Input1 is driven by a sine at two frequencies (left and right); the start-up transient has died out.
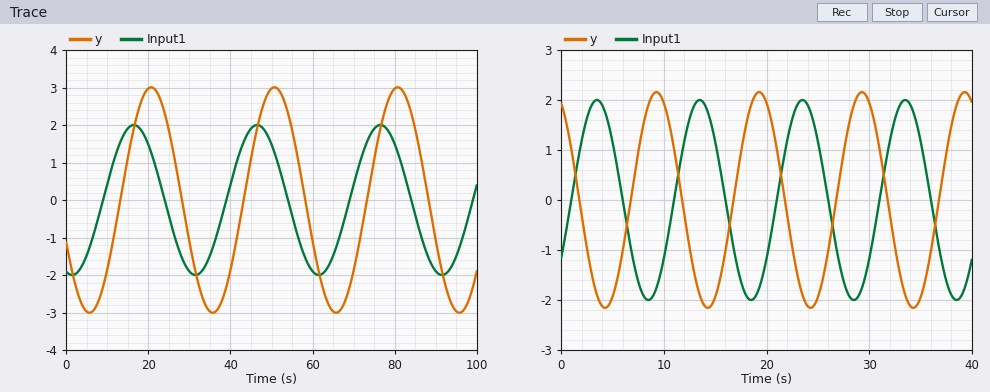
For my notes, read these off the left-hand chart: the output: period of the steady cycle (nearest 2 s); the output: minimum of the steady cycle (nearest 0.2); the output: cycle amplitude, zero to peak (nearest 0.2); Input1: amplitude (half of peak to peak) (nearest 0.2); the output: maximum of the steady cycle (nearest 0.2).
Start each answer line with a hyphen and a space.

- 30 s
- -3.0
- 3.0
- 2.0
- 3.0
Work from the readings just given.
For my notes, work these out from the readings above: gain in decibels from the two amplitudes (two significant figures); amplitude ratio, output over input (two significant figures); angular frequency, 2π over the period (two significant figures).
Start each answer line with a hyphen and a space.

- 3.5 dB
- 1.5
- 0.21 rad/s
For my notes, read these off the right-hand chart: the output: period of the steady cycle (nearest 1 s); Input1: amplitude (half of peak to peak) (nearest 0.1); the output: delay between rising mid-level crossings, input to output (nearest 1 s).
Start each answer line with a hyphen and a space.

- 10 s
- 2.0
- 6 s
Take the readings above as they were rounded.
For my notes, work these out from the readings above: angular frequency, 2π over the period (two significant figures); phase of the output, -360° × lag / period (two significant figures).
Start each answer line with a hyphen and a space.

- 0.63 rad/s
- -220°
